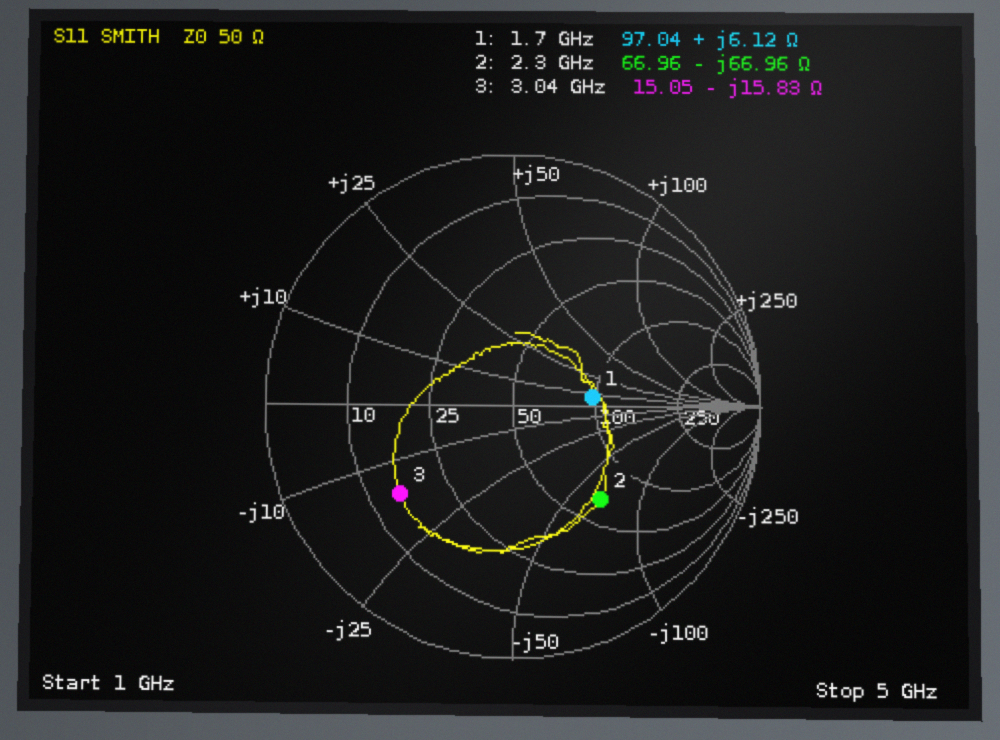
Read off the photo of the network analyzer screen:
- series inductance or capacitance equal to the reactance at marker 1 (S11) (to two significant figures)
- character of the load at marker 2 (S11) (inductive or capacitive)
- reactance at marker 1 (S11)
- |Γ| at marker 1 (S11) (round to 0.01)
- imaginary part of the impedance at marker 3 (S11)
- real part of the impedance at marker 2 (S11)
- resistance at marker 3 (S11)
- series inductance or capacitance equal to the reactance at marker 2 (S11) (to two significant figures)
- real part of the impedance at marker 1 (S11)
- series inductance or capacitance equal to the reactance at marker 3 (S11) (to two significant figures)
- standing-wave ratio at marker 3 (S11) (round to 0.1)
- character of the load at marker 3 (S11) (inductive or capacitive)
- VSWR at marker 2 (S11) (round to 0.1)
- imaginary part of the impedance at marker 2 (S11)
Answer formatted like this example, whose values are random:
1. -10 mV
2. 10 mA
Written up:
1. 570 pH
2. capacitive
3. +6.12 Ω
4. 0.32
5. -15.83 Ω
6. 66.96 Ω
7. 15.05 Ω
8. 1.0 pF
9. 97.04 Ω
10. 3.3 pF
11. 3.7
12. capacitive
13. 3.1
14. -66.96 Ω
